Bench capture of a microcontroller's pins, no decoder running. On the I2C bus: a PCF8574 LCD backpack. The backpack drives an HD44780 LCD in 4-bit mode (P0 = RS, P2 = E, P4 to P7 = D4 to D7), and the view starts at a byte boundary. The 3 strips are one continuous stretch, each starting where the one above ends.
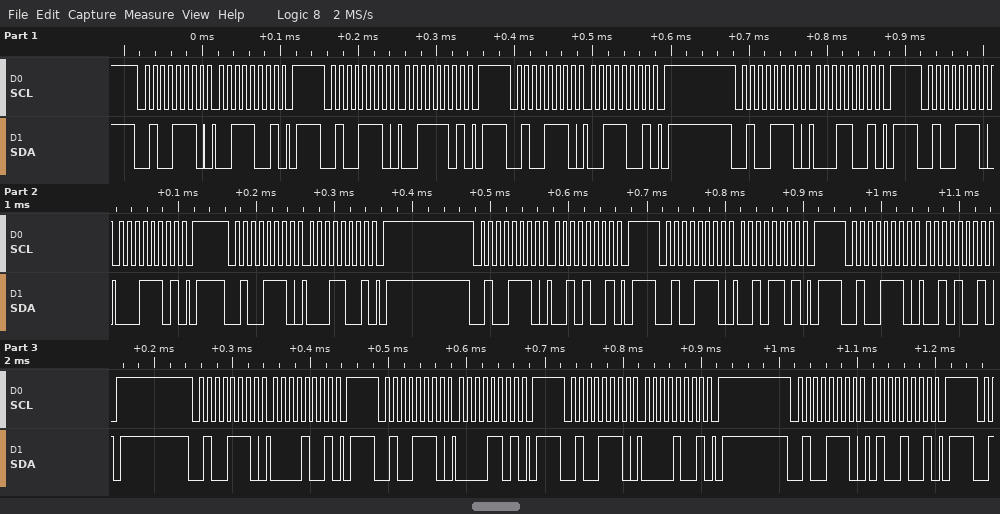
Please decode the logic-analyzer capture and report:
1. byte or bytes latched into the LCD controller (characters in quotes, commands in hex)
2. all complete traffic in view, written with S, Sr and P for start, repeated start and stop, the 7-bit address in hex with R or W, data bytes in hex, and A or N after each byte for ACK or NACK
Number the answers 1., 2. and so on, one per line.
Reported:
1. '1' ' '
2. S 27W A 39 A P S 27W A 3D A P S 27W A 39 A P S 27W A 19 A P S 27W A 1D A P S 27W A 19 A P S 27W A 29 A P S 27W A 2D A P S 27W A 29 A P S 27W A 09 A P S 27W A 0D A P S 27W A 09 A P S 27W A 49 A P
